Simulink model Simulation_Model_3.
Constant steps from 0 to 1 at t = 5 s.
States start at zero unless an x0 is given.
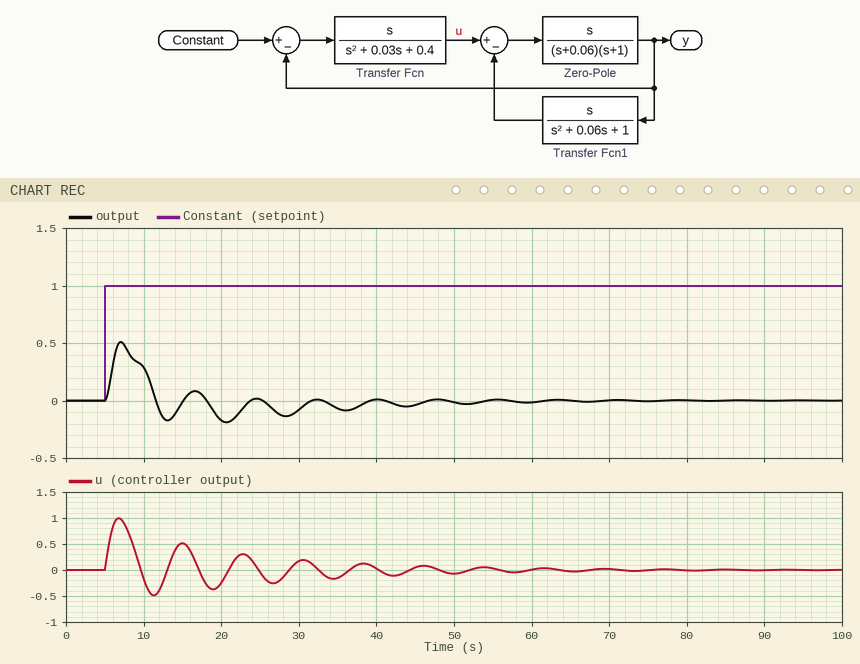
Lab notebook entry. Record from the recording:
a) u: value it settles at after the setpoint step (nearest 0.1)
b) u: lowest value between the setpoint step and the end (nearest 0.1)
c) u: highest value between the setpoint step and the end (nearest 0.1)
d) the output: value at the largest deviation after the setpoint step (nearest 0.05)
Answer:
0.0
-0.5
1.0
0.50
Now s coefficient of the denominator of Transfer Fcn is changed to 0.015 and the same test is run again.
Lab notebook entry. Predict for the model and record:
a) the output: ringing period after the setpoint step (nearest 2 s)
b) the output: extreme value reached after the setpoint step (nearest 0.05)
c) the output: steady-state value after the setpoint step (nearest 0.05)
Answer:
10 s
0.50
0.00
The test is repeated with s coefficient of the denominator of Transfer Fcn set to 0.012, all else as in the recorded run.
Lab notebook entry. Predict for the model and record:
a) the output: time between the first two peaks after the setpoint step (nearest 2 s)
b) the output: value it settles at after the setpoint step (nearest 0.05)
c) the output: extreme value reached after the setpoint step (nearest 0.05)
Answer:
10 s
0.00
0.50
